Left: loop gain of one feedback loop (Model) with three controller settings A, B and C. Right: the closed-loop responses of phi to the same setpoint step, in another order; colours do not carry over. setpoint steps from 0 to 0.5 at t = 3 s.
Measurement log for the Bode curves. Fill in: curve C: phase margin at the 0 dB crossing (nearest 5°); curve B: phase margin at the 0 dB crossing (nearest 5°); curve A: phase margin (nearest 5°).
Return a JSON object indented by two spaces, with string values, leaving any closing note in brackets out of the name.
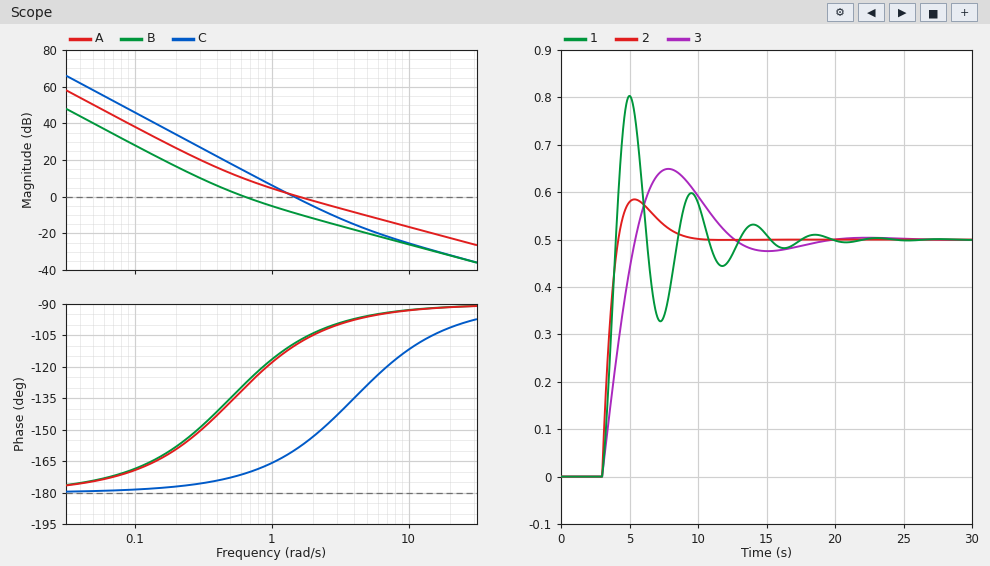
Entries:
{
  "curve C: phase margin at the 0 dB crossing": "20°",
  "curve B: phase margin at the 0 dB crossing": "50°",
  "curve A: phase margin": "70°"
}
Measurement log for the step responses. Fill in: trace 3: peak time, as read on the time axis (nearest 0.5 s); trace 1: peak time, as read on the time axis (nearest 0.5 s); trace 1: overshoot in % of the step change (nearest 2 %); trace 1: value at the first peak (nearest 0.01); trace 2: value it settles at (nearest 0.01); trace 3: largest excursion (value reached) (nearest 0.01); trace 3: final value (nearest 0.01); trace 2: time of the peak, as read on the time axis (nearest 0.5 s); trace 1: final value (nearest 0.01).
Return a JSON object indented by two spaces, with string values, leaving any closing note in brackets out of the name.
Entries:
{
  "trace 3: peak time, as read on the time axis": "8.0 s",
  "trace 1: peak time, as read on the time axis": "5.0 s",
  "trace 1: overshoot in % of the step change": "60 %",
  "trace 1: value at the first peak": "0.80",
  "trace 2: value it settles at": "0.50",
  "trace 3: largest excursion (value reached)": "0.65",
  "trace 3: final value": "0.50",
  "trace 2: time of the peak, as read on the time axis": "5.5 s",
  "trace 1: final value": "0.50"
}
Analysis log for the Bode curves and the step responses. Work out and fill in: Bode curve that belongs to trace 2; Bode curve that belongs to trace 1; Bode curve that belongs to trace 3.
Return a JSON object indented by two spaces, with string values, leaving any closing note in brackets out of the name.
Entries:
{
  "Bode curve that belongs to trace 2": "A",
  "Bode curve that belongs to trace 1": "C",
  "Bode curve that belongs to trace 3": "B"
}
